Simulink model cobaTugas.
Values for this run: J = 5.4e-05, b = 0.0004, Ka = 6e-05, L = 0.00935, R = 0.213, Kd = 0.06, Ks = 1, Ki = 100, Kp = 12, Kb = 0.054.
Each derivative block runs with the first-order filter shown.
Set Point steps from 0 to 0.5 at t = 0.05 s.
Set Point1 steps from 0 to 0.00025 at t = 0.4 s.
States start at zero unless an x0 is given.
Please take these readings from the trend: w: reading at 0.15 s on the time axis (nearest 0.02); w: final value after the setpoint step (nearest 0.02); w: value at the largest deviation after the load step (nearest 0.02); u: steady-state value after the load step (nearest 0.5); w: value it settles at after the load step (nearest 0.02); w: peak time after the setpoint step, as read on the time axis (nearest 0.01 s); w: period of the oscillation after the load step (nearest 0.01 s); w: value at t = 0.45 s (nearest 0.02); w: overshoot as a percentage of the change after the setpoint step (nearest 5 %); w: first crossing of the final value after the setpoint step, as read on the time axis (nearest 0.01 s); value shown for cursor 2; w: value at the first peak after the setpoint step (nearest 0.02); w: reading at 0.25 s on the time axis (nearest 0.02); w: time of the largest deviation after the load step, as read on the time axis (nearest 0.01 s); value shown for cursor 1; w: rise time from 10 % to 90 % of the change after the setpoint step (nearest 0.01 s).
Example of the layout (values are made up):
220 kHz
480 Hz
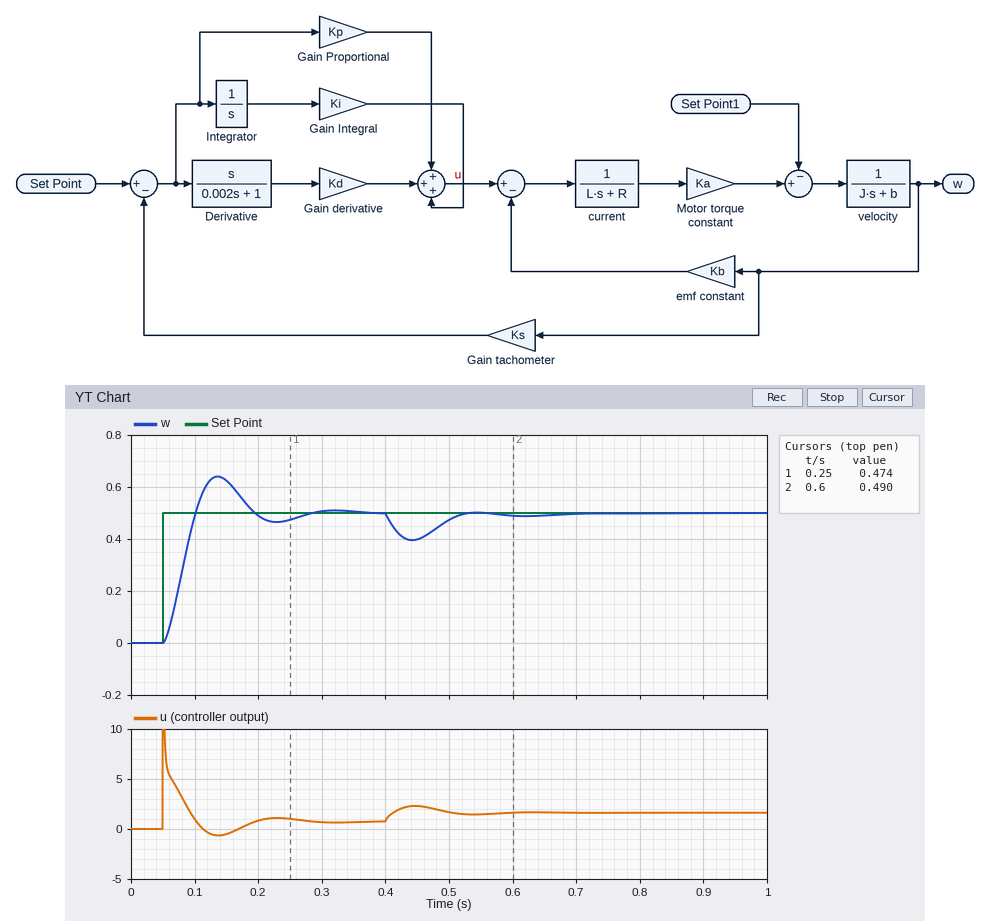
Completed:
0.62
0.50
0.40
1.5
0.50
0.14 s
0.18 s
0.40
30 %
0.10 s
0.490
0.64
0.48
0.44 s
0.474
0.04 s
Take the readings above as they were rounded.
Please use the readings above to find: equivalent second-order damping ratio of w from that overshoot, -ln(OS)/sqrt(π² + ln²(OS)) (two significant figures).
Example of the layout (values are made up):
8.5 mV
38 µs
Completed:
0.36
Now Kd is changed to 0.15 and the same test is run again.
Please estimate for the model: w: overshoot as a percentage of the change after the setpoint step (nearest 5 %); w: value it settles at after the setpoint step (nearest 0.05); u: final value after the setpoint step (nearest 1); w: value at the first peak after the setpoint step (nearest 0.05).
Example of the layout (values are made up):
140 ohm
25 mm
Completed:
15 %
0.50
1
0.60
